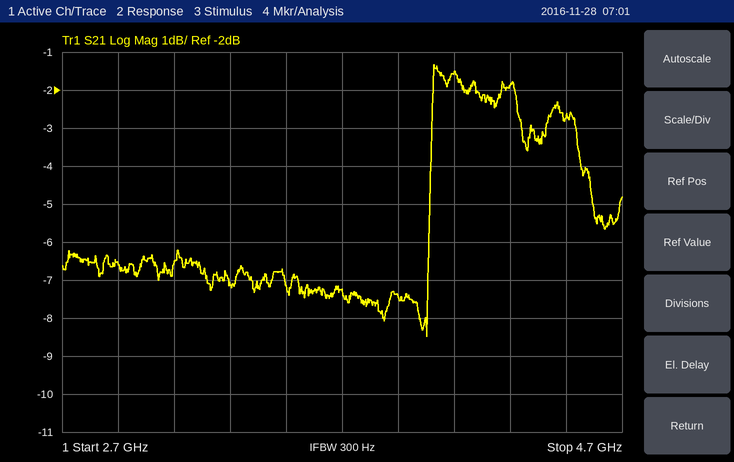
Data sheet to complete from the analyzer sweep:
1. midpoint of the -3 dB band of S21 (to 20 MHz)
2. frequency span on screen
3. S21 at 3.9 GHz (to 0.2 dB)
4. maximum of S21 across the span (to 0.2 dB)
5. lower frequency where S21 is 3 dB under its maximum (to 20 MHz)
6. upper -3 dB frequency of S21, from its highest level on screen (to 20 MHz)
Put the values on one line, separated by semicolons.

4.30 GHz; 2 GHz; -7.4 dB; -1.4 dB; 4.02 GHz; 4.58 GHz
